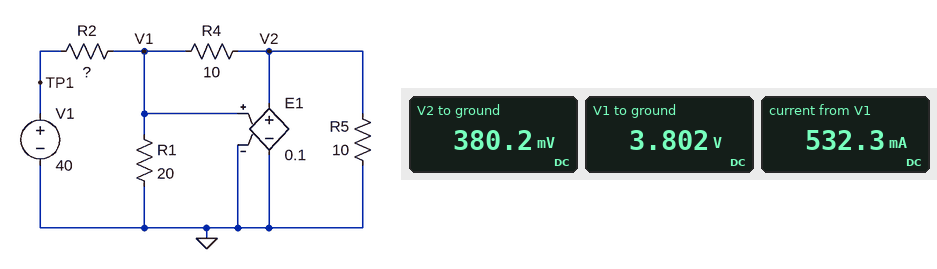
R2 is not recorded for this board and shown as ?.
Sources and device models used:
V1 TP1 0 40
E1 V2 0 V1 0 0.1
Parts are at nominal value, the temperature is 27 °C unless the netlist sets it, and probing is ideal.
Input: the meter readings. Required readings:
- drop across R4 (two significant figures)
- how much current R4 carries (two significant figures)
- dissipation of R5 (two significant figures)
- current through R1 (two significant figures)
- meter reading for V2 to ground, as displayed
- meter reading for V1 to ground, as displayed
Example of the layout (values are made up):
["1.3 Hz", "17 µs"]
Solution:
["3.4 V", "340 mA", "14 mW", "190 mA", "380.2 mV", "3.802 V"]
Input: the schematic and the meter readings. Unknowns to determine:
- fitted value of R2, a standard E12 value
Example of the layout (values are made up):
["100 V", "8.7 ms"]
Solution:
["68 Ω"]
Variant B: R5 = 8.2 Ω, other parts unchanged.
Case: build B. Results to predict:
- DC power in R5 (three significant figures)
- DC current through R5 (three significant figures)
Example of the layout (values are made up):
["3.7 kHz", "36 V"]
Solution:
["17.6 mW", "46.4 mA"]
